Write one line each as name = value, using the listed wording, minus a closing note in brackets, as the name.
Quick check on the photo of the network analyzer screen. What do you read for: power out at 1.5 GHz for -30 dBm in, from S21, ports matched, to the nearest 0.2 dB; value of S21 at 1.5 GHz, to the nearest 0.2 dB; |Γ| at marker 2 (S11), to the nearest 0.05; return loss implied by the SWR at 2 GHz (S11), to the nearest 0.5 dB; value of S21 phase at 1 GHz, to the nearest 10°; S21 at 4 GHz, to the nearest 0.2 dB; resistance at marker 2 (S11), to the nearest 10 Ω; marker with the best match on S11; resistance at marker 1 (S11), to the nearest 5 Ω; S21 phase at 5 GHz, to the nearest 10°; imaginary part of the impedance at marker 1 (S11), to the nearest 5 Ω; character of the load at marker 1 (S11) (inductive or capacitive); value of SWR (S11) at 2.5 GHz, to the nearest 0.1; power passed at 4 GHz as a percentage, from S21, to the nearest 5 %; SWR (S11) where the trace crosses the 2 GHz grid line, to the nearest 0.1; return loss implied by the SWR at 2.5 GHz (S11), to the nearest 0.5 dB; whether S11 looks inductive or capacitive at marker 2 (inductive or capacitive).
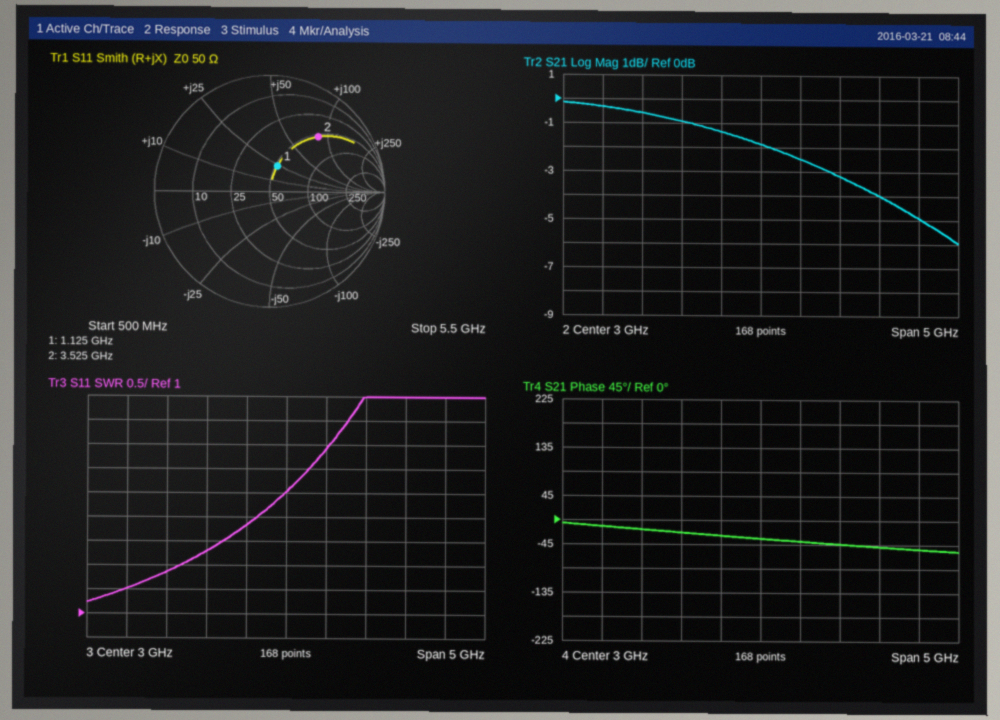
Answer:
power out at 1.5 GHz for -30 dBm in, from S21, ports matched, to the nearest 0.2 dB = -30.6 dBm
value of S21 at 1.5 GHz, to the nearest 0.2 dB = -0.6 dB
|Γ| at marker 2 (S11), to the nearest 0.05 = 0.65
return loss implied by the SWR at 2 GHz (S11), to the nearest 0.5 dB = 8.0 dB
value of S21 phase at 1 GHz, to the nearest 10° = -10°
S21 at 4 GHz, to the nearest 0.2 dB = -3.2 dB
resistance at marker 2 (S11), to the nearest 10 Ω = 50 Ω
marker with the best match on S11 = marker 1
resistance at marker 1 (S11), to the nearest 5 Ω = 50 Ω
S21 phase at 5 GHz, to the nearest 10° = -50°
imaginary part of the impedance at marker 1 (S11), to the nearest 5 Ω = +25 Ω
character of the load at marker 1 (S11) = inductive
value of SWR (S11) at 2.5 GHz, to the nearest 0.1 = 2.8
power passed at 4 GHz as a percentage, from S21, to the nearest 5 % = 50 %
SWR (S11) where the trace crosses the 2 GHz grid line, to the nearest 0.1 = 2.3
return loss implied by the SWR at 2.5 GHz (S11), to the nearest 0.5 dB = 6.5 dB
whether S11 looks inductive or capacitive at marker 2 = inductive
